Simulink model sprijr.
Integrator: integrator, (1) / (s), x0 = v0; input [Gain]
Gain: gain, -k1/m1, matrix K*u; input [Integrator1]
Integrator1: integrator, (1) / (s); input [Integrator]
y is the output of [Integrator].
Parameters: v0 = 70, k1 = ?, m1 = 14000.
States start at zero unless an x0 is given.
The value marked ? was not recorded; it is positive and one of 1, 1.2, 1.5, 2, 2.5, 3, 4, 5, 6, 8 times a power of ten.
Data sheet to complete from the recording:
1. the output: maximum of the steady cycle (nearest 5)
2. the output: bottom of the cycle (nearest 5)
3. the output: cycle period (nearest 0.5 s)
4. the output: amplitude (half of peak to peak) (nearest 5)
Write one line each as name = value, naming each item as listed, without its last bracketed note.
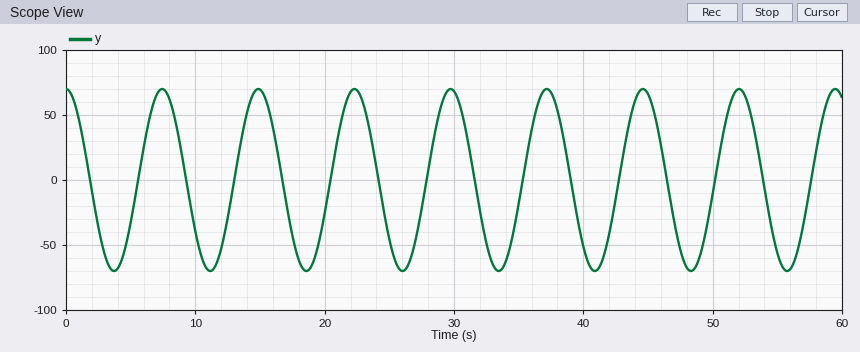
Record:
the output: maximum of the steady cycle = 70
the output: bottom of the cycle = -70
the output: cycle period = 7.5 s
the output: amplitude (half of peak to peak) = 70
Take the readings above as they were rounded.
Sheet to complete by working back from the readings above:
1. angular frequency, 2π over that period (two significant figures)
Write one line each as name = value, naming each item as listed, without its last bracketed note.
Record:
angular frequency, 2π over that period = 0.84 rad/s
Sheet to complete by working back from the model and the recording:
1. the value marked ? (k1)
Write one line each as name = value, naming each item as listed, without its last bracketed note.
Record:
the value marked ? = 10000
